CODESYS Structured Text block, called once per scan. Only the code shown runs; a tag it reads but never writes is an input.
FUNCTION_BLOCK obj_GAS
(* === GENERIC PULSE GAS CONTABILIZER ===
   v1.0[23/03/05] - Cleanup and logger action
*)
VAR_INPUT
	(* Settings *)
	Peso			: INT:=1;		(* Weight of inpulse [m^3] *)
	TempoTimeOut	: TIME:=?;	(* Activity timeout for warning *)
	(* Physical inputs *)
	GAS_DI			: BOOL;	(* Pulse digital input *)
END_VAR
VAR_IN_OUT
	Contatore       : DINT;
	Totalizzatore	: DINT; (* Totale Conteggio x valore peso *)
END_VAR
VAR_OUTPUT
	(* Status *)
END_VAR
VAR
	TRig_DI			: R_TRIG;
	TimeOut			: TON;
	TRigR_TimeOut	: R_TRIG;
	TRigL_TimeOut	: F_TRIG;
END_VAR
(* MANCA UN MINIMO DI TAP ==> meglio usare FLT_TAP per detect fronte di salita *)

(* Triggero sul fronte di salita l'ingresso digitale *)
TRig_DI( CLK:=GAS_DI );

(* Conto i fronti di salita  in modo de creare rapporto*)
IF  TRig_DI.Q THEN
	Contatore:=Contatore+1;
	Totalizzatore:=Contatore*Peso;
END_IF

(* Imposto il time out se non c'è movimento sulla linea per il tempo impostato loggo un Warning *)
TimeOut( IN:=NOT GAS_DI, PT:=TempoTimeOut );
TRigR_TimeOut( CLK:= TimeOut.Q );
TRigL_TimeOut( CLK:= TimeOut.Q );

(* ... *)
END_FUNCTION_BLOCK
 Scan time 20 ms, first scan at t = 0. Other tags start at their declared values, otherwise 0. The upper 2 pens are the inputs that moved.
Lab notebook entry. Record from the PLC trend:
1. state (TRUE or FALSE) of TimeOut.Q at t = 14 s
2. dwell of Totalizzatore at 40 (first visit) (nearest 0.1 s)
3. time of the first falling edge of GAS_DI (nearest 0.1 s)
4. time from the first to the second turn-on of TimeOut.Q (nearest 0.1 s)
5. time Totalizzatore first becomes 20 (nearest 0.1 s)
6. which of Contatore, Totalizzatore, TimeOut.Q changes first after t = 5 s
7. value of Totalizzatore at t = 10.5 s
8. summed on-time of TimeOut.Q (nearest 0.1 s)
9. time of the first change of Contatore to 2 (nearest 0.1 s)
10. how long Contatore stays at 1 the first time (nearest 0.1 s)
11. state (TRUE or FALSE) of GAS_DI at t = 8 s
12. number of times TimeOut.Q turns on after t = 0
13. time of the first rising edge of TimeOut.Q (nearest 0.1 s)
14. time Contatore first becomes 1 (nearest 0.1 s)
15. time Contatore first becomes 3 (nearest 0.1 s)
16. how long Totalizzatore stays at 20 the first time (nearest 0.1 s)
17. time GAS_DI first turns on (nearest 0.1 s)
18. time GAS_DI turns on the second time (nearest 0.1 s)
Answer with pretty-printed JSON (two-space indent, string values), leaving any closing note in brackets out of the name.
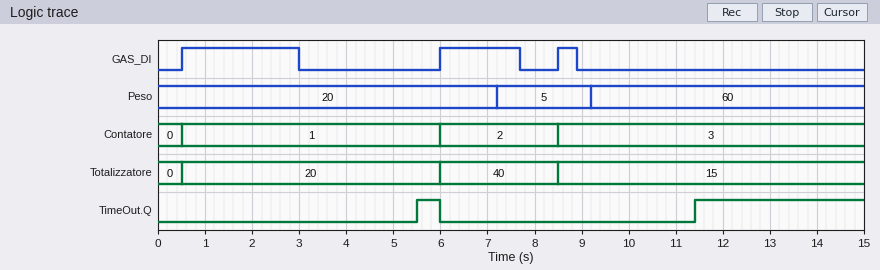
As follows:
{
  "state (TRUE or FALSE) of TimeOut.Q at t = 14 s": "TRUE",
  "dwell of Totalizzatore at 40 (first visit)": "2.5 s",
  "time of the first falling edge of GAS_DI": "3.0 s",
  "time from the first to the second turn-on of TimeOut.Q": "5.9 s",
  "time Totalizzatore first becomes 20": "0.5 s",
  "which of Contatore, Totalizzatore, TimeOut.Q changes first after t = 5 s": "TimeOut.Q",
  "value of Totalizzatore at t = 10.5 s": "15",
  "summed on-time of TimeOut.Q": "4.1 s",
  "time of the first change of Contatore to 2": "6.0 s",
  "how long Contatore stays at 1 the first time": "5.5 s",
  "state (TRUE or FALSE) of GAS_DI at t = 8 s": "FALSE",
  "number of times TimeOut.Q turns on after t = 0": "2",
  "time of the first rising edge of TimeOut.Q": "5.5 s",
  "time Contatore first becomes 1": "0.5 s",
  "time Contatore first becomes 3": "8.5 s",
  "how long Totalizzatore stays at 20 the first time": "5.5 s",
  "time GAS_DI first turns on": "0.5 s",
  "time GAS_DI turns on the second time": "6.0 s"
}
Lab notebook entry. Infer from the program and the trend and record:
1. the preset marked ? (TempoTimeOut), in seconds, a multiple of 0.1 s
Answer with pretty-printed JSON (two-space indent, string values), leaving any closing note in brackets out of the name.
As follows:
{
  "the preset marked ? (TempoTimeOut), in seconds, a multiple of 0.1 s": "2.5 s"
}
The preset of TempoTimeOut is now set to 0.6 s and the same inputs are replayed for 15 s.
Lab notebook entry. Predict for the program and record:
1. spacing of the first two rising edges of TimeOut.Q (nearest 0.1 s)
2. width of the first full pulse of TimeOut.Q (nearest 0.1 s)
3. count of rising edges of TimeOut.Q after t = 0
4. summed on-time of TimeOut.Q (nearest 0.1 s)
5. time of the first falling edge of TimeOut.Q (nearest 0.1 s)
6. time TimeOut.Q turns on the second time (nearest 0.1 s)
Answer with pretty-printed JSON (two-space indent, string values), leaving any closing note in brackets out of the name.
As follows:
{
  "spacing of the first two rising edges of TimeOut.Q": "4.7 s",
  "width of the first full pulse of TimeOut.Q": "2.4 s",
  "count of rising edges of TimeOut.Q after t = 0": "3",
  "summed on-time of TimeOut.Q": "8.1 s",
  "time of the first falling edge of TimeOut.Q": "6.0 s",
  "time TimeOut.Q turns on the second time": "8.3 s"
}
